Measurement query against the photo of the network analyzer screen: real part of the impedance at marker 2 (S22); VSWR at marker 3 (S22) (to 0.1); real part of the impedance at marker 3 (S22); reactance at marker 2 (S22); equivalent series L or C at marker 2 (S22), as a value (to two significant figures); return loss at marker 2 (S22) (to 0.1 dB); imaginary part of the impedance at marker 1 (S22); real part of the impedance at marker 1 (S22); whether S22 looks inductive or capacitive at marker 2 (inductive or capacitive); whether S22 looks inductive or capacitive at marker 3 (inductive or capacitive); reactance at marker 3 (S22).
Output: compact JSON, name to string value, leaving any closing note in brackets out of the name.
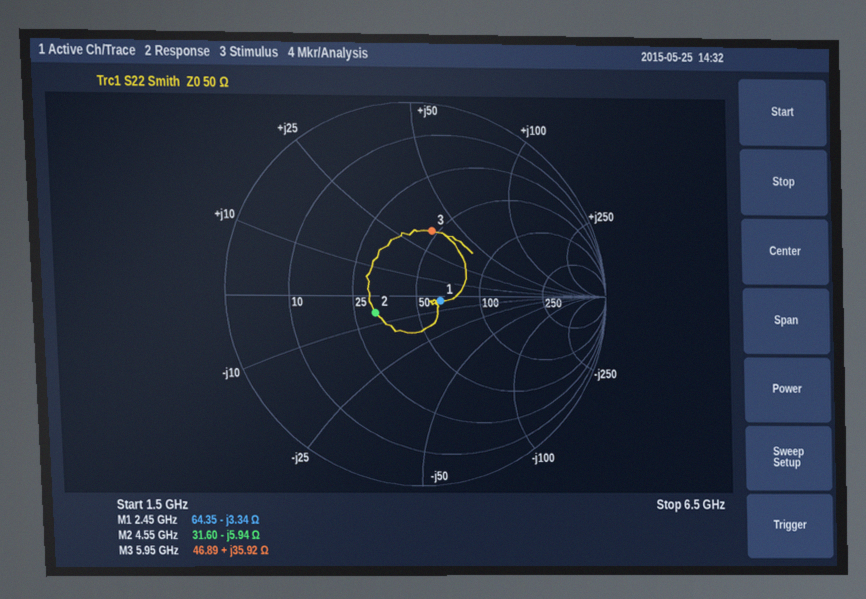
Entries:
{"real part of the impedance at marker 2": "31.60 Ω", "VSWR at marker 3 (S22)": "2.1", "real part of the impedance at marker 3": "46.89 Ω", "reactance at marker 2": "-5.94 Ω", "equivalent series L or C at marker 2 (S22), as a value": "5.9 pF", "return loss at marker 2 (S22)": "12.5 dB", "imaginary part of the impedance at marker 1": "-3.34 Ω", "real part of the impedance at marker 1": "64.35 Ω", "whether S22 looks inductive or capacitive at marker 2": "capacitive", "whether S22 looks inductive or capacitive at marker 3": "inductive", "reactance at marker 3": "+35.92 Ω"}
